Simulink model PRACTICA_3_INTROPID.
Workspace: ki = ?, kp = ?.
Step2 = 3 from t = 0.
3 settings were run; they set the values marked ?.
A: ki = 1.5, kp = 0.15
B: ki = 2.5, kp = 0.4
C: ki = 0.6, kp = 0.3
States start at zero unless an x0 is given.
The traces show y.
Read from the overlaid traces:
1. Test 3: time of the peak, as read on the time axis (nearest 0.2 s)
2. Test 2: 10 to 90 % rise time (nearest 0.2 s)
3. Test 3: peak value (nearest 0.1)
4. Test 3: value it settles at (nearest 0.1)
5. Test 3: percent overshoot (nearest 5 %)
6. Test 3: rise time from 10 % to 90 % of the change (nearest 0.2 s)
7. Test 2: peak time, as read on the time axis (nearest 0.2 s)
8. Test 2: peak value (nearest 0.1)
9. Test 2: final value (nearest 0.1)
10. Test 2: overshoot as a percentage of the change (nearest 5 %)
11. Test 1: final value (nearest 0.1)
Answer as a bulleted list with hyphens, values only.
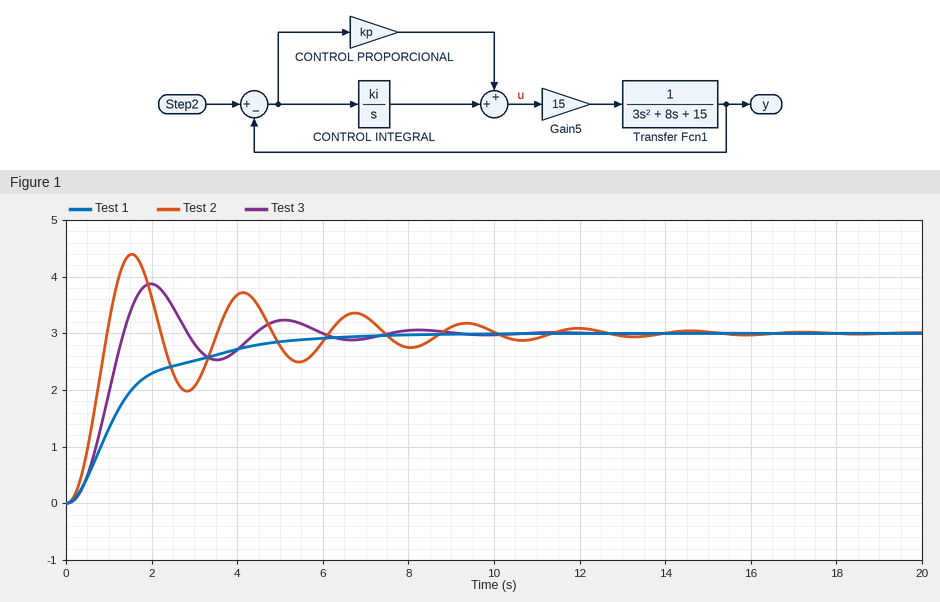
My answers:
- 2.0 s
- 0.6 s
- 3.9
- 3.0
- 30 %
- 0.8 s
- 1.6 s
- 4.4
- 3.0
- 45 %
- 3.0
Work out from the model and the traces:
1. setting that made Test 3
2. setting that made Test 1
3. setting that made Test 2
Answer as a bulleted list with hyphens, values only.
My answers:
- A
- C
- B
